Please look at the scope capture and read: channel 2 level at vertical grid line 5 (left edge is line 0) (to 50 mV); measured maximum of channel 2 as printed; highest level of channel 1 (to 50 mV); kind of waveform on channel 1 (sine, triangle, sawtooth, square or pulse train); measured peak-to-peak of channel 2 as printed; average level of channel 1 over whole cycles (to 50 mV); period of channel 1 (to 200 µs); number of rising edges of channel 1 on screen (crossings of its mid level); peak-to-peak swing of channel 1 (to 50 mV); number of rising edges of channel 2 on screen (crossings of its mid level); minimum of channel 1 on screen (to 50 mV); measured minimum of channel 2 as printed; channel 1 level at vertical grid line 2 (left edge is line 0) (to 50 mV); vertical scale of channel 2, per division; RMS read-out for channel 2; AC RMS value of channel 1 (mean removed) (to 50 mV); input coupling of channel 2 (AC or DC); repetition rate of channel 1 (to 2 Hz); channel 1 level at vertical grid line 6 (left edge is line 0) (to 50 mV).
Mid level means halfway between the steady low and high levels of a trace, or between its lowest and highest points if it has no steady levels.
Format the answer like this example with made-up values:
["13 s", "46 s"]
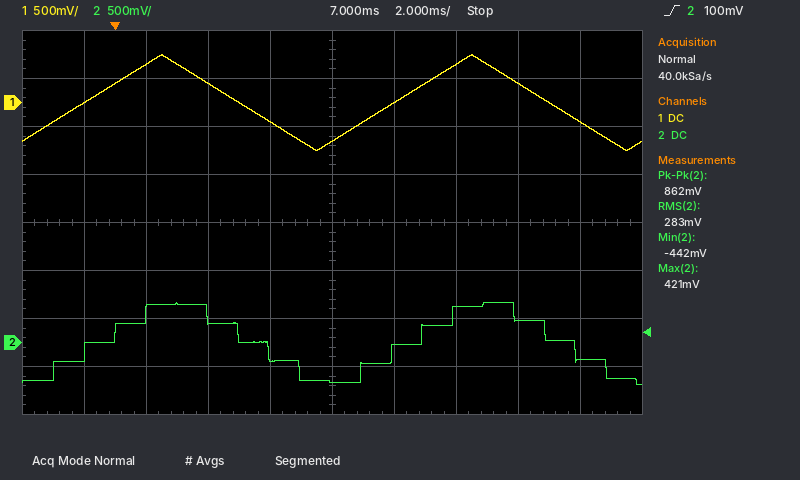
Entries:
["-400 mV", "421 mV", "500 mV", "triangle", "862 mV", "0 mV", "10.0 ms", "2", "1.00 V", "2", "-500 mV", "-442 mV", "400 mV", "500 mV", "283 mV", "300 mV", "DC", "100 Hz", "0 mV"]
